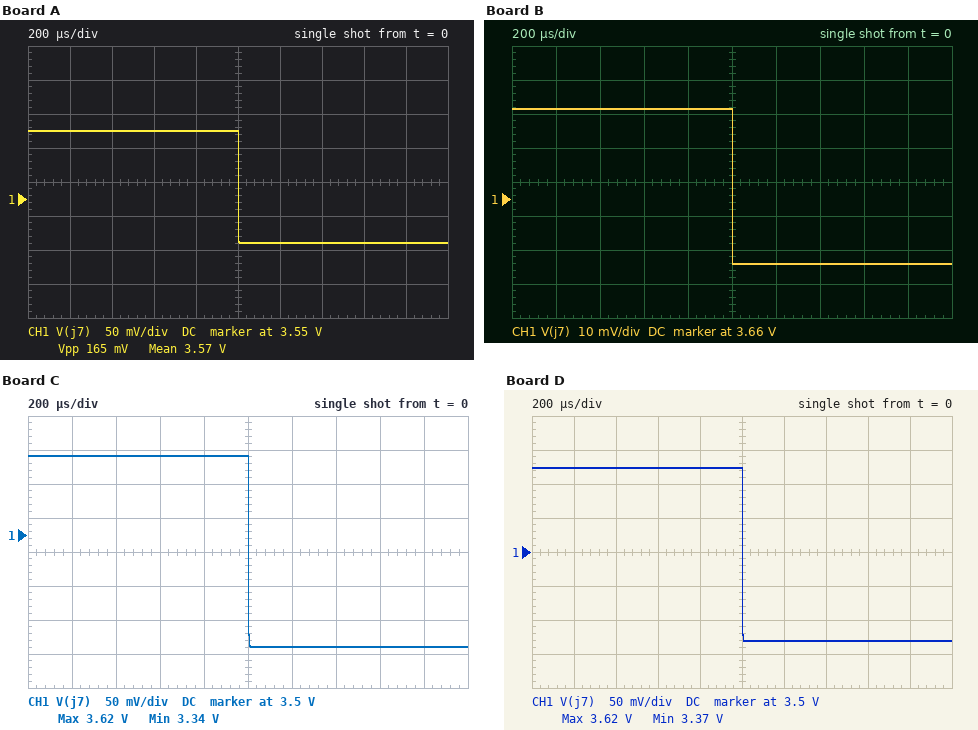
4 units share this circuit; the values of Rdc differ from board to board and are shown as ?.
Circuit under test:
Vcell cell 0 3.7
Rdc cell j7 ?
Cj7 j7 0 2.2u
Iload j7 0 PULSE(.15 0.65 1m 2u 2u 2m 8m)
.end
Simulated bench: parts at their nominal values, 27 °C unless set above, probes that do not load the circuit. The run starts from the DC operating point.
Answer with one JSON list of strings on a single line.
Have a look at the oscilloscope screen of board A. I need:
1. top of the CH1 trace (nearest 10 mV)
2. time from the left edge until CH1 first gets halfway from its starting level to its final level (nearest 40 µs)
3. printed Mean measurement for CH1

["3.65 V", "1.00 ms", "3.57 V"]
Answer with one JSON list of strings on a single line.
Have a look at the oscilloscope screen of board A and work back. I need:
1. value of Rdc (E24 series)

["0.33 Ω"]
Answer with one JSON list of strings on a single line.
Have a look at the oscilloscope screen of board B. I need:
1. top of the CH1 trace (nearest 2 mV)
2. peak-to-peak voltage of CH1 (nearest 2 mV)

["3.686 V", "46 mV"]
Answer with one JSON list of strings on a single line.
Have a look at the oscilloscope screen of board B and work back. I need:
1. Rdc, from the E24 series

["0.091 Ω"]
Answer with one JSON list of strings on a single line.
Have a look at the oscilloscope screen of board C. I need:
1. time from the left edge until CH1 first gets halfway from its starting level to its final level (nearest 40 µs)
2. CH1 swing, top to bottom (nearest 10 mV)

["1.00 ms", "280 mV"]
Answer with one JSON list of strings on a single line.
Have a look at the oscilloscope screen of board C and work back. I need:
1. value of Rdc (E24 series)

["0.56 Ω"]
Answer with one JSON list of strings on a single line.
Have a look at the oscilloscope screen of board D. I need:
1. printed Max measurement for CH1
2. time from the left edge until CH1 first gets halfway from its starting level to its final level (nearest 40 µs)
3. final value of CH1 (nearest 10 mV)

["3.62 V", "1.00 ms", "3.37 V"]
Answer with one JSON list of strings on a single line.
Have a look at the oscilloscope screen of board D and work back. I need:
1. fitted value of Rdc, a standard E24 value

["0.51 Ω"]
